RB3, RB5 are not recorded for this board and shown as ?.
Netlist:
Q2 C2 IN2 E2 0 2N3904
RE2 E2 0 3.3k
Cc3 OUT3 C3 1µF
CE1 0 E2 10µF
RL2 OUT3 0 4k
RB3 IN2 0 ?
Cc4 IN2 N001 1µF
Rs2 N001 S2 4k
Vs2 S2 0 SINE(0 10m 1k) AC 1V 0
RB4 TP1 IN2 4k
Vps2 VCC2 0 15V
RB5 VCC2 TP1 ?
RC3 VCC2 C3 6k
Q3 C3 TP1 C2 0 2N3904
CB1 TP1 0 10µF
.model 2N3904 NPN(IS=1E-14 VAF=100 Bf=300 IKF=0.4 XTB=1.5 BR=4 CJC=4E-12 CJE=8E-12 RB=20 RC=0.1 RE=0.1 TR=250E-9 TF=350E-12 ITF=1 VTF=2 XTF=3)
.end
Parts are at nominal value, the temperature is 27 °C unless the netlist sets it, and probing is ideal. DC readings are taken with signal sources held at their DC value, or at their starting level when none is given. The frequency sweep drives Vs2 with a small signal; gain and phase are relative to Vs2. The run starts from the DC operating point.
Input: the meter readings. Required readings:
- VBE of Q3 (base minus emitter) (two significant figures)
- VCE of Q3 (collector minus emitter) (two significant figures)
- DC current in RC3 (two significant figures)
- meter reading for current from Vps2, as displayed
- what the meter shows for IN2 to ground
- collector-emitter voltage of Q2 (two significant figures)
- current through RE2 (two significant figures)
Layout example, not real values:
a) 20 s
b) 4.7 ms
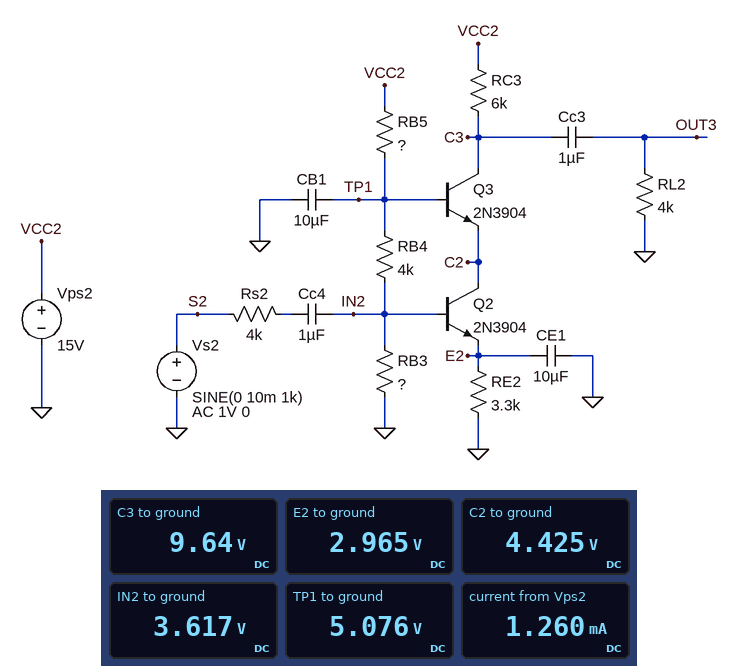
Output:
a) 650 mV
b) 5.2 V
c) 890 µA
d) 1.260 mA
e) 3.617 V
f) 1.5 V
g) 900 µA
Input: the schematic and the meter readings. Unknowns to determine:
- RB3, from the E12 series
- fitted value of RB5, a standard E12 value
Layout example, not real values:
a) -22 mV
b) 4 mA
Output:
a) 10 kΩ
b) 27 kΩ
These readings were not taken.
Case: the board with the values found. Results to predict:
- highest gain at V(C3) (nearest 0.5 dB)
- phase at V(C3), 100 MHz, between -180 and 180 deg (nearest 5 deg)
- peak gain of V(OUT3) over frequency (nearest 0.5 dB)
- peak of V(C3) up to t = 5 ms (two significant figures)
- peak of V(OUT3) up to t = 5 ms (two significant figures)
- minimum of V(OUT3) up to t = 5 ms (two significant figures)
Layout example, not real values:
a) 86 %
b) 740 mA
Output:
a) 29.0 dB
b) -10 deg
c) 29.0 dB
d) 9.9 V
e) 270 mV
f) -270 mV
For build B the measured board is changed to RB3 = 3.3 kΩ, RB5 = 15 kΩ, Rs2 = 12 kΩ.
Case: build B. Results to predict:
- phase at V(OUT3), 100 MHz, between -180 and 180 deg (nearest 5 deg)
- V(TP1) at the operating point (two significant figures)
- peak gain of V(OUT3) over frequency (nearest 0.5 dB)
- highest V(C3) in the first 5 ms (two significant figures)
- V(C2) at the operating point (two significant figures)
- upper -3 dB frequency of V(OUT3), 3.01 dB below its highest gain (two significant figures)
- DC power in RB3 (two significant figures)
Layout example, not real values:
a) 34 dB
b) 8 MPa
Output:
a) -15 deg
b) 4.9 V
c) 14.5 dB
d) 12 V
e) 4.3 V
f) 4.5 MHz
g) 1.5 mW
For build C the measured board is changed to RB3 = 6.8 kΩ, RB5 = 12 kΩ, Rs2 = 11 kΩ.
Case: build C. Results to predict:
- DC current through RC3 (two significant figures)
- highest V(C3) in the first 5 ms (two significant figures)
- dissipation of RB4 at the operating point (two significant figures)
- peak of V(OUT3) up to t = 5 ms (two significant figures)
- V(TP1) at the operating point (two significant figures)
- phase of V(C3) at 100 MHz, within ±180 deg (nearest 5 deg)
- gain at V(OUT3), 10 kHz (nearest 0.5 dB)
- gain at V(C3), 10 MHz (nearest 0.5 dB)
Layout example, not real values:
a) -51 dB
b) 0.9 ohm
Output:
a) 1.1 mA
b) 8.3 V
c) 1.7 mW
d) 140 mV
e) 7.1 V
f) -10 deg
g) 23.5 dB
h) 12.0 dB
